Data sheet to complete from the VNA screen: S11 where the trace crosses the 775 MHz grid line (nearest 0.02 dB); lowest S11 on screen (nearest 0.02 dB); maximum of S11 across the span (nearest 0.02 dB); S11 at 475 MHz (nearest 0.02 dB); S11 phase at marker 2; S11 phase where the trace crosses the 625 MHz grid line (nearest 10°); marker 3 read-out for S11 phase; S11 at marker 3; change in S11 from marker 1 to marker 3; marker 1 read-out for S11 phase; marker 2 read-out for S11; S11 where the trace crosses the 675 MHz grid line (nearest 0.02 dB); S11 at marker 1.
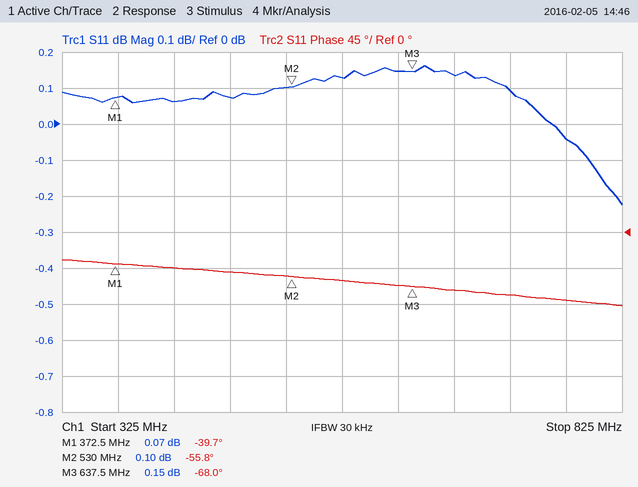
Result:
-0.04 dB
-0.22 dB
0.16 dB
0.08 dB
-55.8°
-70°
-68.0°
0.15 dB
0.08 dB
-39.7°
0.10 dB
0.14 dB
0.07 dB
